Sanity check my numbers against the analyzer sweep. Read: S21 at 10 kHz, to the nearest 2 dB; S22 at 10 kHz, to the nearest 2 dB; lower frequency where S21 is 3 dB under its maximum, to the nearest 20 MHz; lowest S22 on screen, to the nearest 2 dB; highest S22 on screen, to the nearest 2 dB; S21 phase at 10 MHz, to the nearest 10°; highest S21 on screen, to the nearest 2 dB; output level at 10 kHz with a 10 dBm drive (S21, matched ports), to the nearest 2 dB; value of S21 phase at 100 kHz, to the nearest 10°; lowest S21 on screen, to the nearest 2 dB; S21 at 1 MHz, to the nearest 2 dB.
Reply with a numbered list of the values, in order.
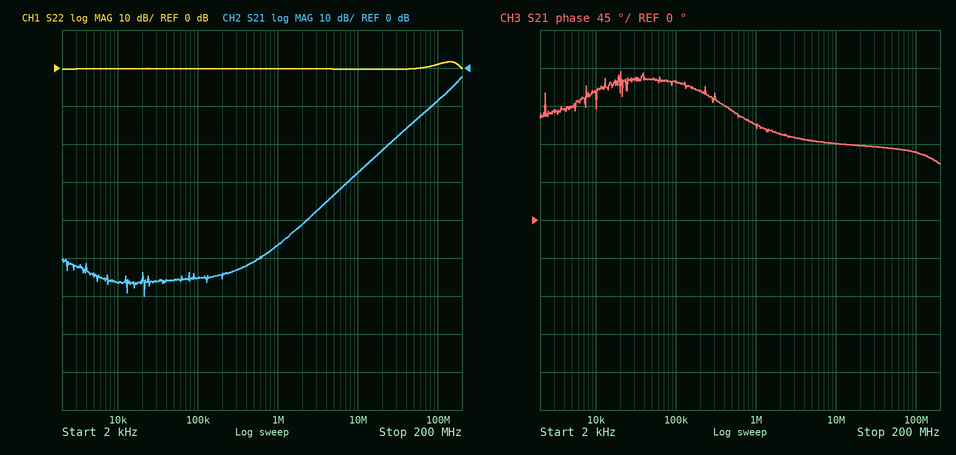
1. -56 dB
2. 0 dB
3. 140 MHz
4. 0 dB
5. 2 dB
6. 90°
7. -2 dB
8. -46 dBm
9. 160°
10. -60 dB
11. -46 dB
